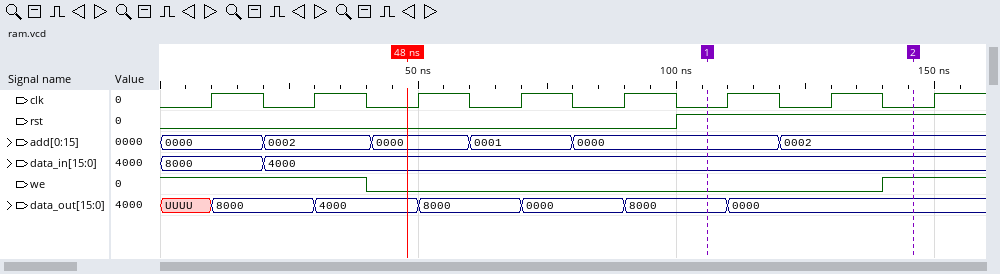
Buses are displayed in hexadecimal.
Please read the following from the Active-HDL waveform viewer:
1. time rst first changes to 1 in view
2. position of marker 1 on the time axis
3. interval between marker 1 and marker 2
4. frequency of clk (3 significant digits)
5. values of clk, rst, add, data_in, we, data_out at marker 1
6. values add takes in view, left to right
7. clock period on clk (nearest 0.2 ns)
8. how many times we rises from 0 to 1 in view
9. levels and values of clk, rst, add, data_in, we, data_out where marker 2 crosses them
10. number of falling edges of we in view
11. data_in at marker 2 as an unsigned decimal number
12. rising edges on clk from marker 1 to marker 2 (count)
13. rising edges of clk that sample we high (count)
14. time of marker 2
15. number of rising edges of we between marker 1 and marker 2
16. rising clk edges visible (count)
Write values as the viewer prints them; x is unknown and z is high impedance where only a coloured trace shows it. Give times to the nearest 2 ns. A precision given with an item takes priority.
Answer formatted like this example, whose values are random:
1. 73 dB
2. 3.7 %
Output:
1. 100 ns
2. 106 ns
3. 40 ns
4. 50.0 MHz
5. clk=0, rst=1, add=0000, data_in=4000, we=0, data_out=8000
6. 0000, 0002, 0000, 0001, 0000, 0002
7. 20 ns
8. 1
9. clk=0, rst=1, add=0002, data_in=4000, we=1, data_out=0000
10. 1
11. 16384
12. 2
13. 3
14. 146 ns
15. 1
16. 8
